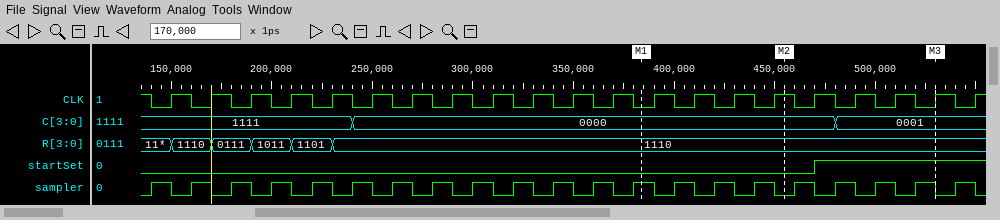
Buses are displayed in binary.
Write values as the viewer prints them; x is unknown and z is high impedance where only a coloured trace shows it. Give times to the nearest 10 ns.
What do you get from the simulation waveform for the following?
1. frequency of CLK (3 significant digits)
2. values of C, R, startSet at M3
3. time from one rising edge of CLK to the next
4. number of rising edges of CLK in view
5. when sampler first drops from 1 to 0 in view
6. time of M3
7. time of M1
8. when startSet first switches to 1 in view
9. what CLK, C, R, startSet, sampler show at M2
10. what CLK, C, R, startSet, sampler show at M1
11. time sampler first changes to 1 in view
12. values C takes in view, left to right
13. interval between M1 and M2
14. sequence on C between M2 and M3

50.0 MHz
C=0001, R=1110, startSet=1
20 ns
21
150 ns
530 ns
380 ns
470 ns
CLK=1, C=0000, R=1110, startSet=0, sampler=0
CLK=0, C=0000, R=1110, startSet=0, sampler=1
140 ns
1111, 0000, 0001
70 ns
0000, 0001
